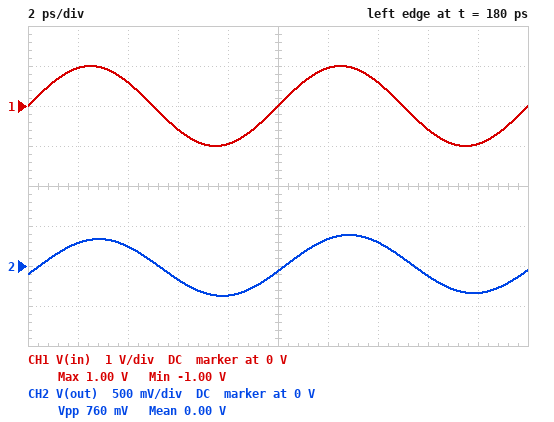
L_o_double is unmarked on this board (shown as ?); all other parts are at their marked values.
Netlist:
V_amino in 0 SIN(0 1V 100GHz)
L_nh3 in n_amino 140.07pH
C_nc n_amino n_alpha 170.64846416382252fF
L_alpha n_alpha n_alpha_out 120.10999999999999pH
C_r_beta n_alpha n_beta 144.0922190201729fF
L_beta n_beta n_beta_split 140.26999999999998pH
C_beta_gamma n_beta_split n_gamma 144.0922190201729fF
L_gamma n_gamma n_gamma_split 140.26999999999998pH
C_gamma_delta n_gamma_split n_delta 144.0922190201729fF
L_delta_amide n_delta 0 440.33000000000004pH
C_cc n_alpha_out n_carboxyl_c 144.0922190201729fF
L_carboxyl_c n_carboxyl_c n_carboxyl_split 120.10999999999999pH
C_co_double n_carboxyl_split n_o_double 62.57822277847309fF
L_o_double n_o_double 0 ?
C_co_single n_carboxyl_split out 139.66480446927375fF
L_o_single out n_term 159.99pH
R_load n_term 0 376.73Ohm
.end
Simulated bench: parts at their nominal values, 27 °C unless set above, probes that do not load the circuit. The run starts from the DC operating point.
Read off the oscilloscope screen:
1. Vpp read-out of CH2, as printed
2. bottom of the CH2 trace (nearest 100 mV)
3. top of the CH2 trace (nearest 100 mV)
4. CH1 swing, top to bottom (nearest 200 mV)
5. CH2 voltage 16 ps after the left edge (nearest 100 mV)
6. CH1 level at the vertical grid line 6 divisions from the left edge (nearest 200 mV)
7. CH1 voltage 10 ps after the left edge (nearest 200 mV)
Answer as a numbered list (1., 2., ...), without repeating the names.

1. 760 mV
2. -400 mV
3. 400 mV
4. 2.0 V
5. -100 mV
6. 1.0 V
7. 0 V
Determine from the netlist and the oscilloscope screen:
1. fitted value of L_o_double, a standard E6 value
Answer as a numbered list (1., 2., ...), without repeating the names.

1. 330 pH
